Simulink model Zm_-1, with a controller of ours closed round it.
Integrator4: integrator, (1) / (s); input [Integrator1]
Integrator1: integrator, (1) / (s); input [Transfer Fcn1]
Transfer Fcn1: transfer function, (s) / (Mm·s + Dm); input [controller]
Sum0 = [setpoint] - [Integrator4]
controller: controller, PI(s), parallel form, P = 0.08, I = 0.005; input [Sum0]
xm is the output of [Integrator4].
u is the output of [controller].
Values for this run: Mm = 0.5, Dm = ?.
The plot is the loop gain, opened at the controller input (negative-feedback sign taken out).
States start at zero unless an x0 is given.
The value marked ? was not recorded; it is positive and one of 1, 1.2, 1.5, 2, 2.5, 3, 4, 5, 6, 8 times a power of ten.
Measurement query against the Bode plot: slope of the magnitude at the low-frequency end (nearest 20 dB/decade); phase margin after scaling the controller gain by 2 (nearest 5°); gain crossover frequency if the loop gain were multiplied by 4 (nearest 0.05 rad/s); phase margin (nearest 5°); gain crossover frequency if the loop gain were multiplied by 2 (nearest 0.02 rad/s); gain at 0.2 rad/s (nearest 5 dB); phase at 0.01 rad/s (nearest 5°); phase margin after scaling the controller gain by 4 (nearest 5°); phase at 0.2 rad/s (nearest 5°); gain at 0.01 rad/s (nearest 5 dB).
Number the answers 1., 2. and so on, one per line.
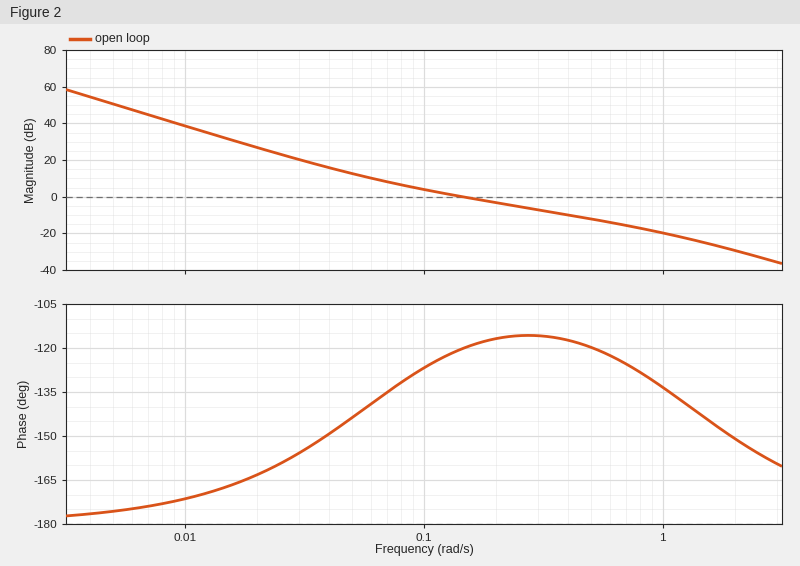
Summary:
1. -40 dB/decade
2. 65°
3. 0.50 rad/s
4. 60°
5. 0.26 rad/s
6. -5 dB
7. -170°
8. 60°
9. -115°
10. 40 dB
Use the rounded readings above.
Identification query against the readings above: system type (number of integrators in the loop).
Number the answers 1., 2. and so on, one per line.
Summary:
1. 2
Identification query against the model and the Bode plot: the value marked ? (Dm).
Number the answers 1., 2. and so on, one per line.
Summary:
1. 0.6
